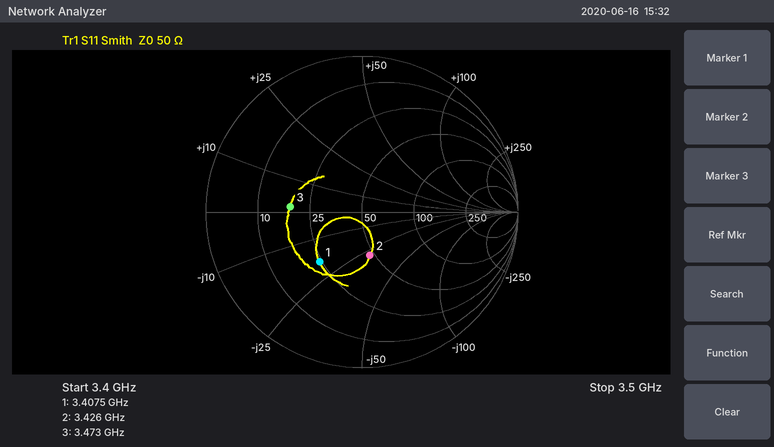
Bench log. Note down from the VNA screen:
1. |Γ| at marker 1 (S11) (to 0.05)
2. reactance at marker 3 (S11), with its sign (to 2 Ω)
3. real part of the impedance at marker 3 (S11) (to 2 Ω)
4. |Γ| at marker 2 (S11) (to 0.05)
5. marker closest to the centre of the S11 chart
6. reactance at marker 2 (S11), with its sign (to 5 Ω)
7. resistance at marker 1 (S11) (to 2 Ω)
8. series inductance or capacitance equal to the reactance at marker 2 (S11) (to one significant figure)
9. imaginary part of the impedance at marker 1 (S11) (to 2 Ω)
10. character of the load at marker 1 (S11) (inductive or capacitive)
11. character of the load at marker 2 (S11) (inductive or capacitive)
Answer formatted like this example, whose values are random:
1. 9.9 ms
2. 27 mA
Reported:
1. 0.40
2. +2 Ω
3. 18 Ω
4. 0.30
5. marker 2
6. -30 Ω
7. 24 Ω
8. 2 pF
9. -18 Ω
10. capacitive
11. capacitive
